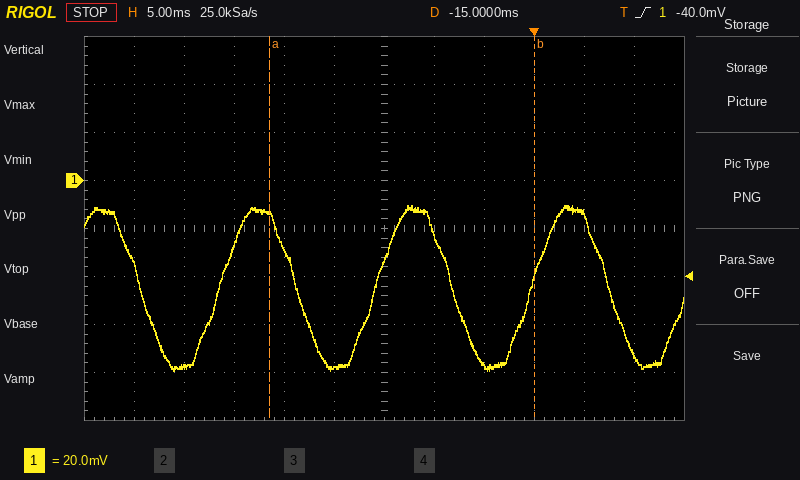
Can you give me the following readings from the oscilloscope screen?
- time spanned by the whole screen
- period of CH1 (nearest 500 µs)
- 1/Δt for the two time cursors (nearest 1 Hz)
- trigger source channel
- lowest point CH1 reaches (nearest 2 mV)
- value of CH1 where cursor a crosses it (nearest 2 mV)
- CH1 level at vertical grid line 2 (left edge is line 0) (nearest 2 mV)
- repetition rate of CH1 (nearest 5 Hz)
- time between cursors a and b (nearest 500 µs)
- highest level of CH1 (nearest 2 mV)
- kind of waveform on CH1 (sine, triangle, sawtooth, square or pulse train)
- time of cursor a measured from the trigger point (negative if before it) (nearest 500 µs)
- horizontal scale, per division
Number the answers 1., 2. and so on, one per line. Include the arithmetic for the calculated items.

1. 60 ms
2. 15.5 ms
3. 1 / 26.5 ms ≈ 38 Hz
4. CH1
5. -80 mV
6. -14 mV
7. -78 mV
8. 1 / 15.5 ms ≈ 65 Hz
9. 26.5 ms
10. -10 mV
11. sine
12. -26.5 ms
13. 5 ms
